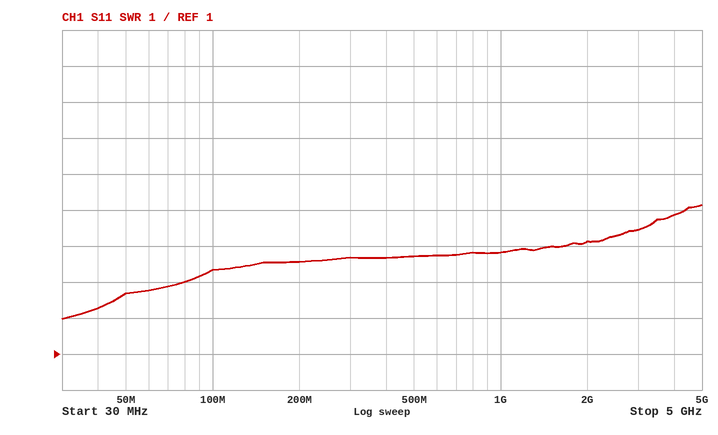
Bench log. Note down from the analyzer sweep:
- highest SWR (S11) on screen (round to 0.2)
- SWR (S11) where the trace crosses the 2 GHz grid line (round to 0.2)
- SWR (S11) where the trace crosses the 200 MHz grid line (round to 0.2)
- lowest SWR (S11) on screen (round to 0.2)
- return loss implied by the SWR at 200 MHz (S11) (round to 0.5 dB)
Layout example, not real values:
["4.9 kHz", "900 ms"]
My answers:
["5.2", "4.2", "3.6", "2.0", "5.0 dB"]
